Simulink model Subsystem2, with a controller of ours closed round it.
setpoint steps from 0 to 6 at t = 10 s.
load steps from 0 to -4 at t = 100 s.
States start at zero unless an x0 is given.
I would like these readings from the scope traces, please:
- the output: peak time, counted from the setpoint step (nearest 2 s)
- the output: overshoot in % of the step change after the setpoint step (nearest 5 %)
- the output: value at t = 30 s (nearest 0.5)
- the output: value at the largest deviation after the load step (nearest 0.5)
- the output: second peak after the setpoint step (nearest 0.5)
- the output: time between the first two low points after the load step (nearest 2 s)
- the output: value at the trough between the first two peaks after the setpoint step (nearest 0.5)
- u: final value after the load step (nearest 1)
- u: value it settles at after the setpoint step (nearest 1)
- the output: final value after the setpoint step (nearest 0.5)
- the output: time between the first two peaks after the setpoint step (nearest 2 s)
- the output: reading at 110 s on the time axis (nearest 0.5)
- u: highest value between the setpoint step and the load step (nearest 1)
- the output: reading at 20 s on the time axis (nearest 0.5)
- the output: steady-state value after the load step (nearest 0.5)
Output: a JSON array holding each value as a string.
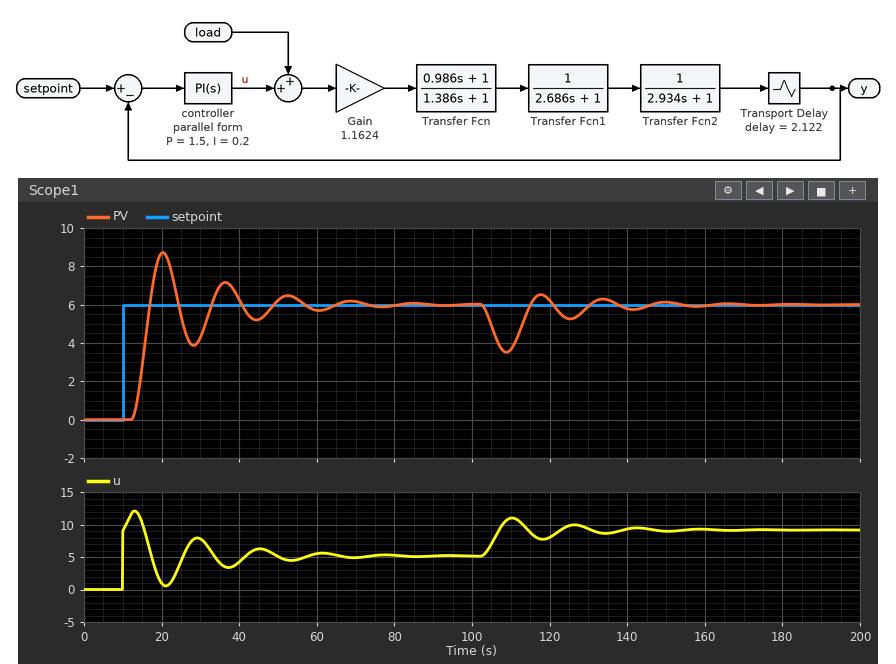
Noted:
["10 s", "45 %", "4.5", "3.5", "7.0", "16 s", "4.0", "9", "5", "6.0", "16 s", "3.5", "12", "8.5", "6.0"]
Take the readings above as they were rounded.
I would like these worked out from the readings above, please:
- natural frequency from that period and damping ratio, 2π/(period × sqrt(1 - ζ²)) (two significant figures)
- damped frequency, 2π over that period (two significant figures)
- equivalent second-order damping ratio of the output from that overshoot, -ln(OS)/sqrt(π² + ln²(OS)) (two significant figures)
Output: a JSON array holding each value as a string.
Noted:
["0.41 rad/s", "0.39 rad/s", "0.25"]
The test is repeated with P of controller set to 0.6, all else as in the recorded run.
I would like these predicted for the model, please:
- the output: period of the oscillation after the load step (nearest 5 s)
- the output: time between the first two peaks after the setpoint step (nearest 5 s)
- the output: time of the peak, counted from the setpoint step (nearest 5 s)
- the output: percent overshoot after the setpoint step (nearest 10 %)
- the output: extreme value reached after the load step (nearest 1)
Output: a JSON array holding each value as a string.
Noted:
["25 s", "25 s", "15 s", "40 %", "3"]
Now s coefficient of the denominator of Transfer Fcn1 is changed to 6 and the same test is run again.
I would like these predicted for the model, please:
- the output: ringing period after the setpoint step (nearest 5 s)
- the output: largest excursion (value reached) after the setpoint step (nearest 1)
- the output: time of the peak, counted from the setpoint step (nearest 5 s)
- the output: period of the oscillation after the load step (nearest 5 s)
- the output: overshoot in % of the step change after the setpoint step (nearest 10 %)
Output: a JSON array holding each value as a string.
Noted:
["25 s", "9", "15 s", "25 s", "40 %"]
